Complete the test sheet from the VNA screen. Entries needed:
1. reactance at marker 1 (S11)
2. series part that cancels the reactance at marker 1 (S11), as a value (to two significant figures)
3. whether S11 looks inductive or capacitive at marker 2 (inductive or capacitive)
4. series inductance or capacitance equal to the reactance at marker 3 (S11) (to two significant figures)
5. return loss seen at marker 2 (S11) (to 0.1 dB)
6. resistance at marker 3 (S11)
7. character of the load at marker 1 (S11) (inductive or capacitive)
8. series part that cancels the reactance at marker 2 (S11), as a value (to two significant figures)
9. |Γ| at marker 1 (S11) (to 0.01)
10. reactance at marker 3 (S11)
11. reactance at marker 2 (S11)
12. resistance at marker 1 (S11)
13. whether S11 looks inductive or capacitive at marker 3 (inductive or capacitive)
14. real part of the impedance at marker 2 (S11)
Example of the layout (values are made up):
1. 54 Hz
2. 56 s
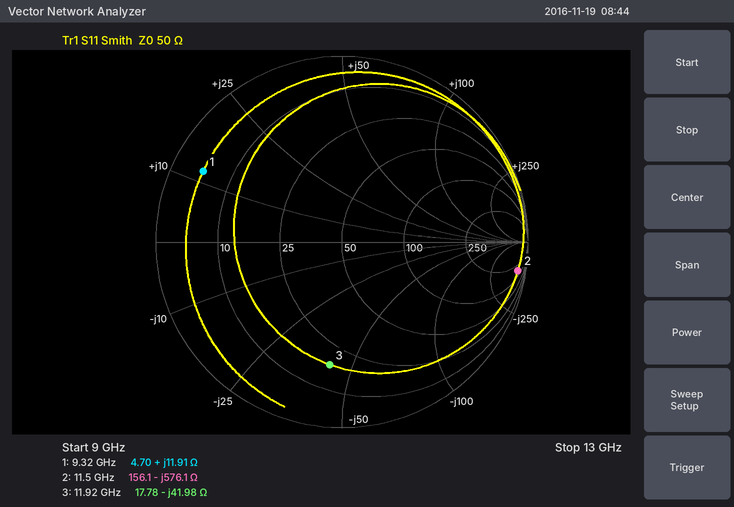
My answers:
1. +11.91 Ω
2. 1.4 pF
3. capacitive
4. 320 fF
5. 0.4 dB
6. 17.78 Ω
7. inductive
8. 8.0 nH
9. 0.84
10. -41.98 Ω
11. -576.1 Ω
12. 4.70 Ω
13. capacitive
14. 156.1 Ω
